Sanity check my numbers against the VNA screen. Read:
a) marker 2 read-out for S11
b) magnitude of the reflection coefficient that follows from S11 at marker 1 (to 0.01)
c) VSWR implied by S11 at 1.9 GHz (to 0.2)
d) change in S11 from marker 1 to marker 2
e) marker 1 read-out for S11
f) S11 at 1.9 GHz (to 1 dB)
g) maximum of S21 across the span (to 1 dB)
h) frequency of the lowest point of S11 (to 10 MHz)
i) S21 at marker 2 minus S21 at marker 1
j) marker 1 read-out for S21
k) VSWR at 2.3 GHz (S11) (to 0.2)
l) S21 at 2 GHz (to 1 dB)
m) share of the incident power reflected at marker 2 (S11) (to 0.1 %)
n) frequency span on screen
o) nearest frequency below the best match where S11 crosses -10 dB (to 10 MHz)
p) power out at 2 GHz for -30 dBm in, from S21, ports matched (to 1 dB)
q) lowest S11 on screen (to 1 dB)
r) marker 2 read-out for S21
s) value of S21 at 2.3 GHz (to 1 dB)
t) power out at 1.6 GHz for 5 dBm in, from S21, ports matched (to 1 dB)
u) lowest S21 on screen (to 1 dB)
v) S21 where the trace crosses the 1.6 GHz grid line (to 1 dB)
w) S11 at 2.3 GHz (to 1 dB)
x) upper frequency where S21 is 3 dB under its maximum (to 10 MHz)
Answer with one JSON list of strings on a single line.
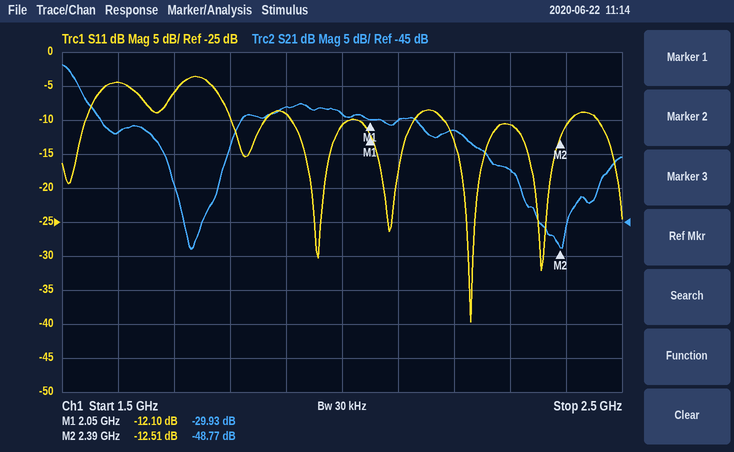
["-12.51 dB", "0.25", "2.0", "-0.41 dB", "-12.10 dB", "-9 dB", "-22 dB", "2.23 GHz", "-18.84 dB", "-29.93 dB", "1.8", "-29 dB", "5.6 %", "1 GHz", "2.18 GHz", "-59 dBm", "-40 dB", "-48.77 dB", "-37 dB", "-27 dBm", "-49 dB", "-32 dB", "-11 dB", "1.53 GHz"]
